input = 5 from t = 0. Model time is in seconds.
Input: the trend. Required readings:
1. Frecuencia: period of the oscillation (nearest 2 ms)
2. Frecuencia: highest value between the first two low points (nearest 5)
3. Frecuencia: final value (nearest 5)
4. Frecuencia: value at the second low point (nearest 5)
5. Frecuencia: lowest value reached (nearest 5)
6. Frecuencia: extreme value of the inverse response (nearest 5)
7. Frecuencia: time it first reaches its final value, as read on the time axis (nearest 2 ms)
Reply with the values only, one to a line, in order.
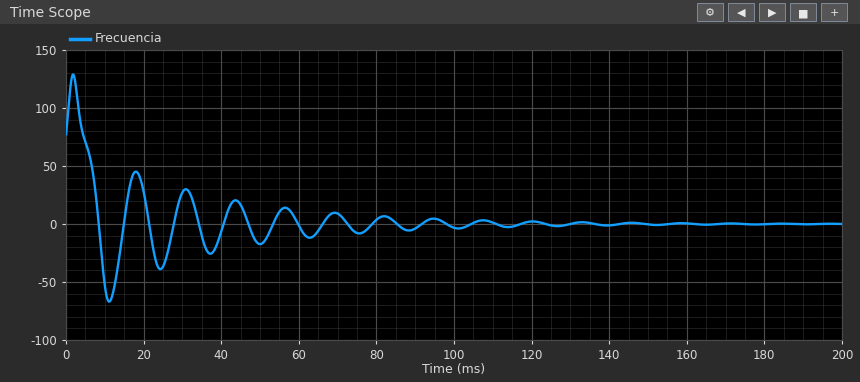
14 ms
45
0
-40
-65
130
8 ms
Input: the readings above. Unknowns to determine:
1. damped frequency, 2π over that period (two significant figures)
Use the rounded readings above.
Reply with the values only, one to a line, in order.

0.45 rad/ms
